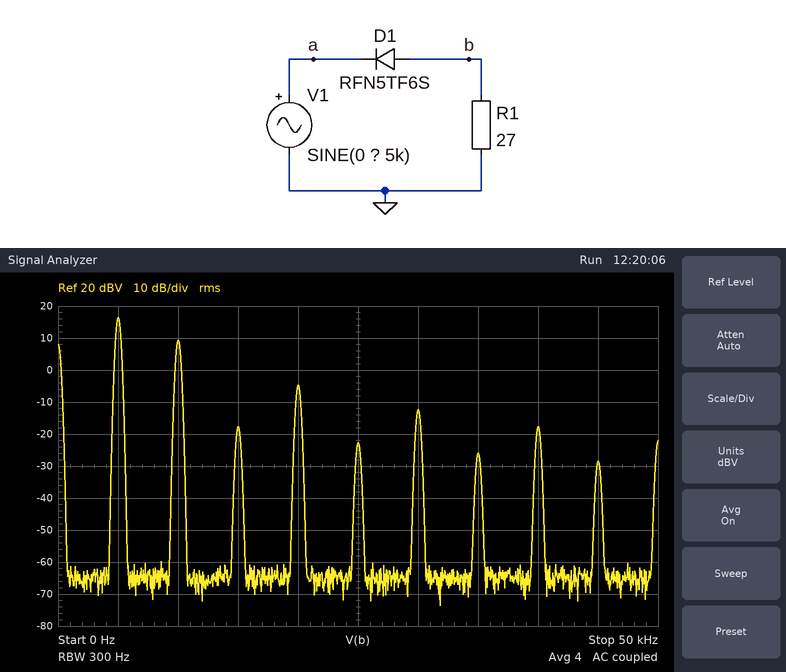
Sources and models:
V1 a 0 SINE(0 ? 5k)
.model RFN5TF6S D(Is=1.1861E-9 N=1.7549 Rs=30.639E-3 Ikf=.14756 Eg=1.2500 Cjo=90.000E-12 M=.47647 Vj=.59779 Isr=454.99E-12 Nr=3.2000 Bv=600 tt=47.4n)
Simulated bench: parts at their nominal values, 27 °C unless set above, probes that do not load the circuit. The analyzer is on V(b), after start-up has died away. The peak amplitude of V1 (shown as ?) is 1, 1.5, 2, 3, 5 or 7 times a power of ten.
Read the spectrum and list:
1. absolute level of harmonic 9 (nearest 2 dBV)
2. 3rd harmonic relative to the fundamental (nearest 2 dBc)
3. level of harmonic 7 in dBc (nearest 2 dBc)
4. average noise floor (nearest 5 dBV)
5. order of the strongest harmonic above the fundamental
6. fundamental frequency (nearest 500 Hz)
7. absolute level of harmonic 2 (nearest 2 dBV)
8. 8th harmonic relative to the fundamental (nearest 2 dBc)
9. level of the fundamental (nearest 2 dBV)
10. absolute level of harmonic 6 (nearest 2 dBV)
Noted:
-28 dBV
-34 dBc
-42 dBc
-65 dBV
2
5.0 kHz
10 dBV
-34 dBc
16 dBV
-12 dBV
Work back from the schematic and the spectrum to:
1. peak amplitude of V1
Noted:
20 V
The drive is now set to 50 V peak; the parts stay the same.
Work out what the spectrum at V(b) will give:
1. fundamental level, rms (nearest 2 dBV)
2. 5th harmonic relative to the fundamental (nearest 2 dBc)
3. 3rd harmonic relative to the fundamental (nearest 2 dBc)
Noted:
24 dBV
-46 dBc
-42 dBc
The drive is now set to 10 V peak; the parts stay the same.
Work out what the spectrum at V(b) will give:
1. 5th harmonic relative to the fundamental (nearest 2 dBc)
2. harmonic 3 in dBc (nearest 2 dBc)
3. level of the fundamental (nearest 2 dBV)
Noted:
-34 dBc
-28 dBc
10 dBV
